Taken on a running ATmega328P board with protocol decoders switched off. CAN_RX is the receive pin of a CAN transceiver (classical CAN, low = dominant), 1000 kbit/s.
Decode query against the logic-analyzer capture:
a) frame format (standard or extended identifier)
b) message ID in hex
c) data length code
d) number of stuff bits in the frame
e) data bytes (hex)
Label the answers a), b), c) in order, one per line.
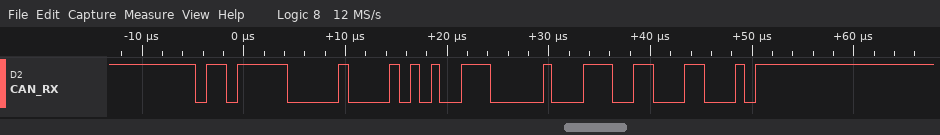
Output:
a) standard
b) 0x6F8
c) 2
d) 3
e) A7 00
